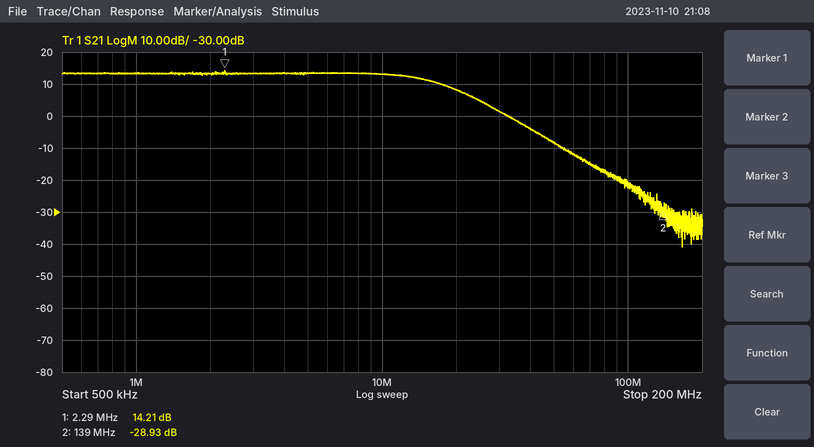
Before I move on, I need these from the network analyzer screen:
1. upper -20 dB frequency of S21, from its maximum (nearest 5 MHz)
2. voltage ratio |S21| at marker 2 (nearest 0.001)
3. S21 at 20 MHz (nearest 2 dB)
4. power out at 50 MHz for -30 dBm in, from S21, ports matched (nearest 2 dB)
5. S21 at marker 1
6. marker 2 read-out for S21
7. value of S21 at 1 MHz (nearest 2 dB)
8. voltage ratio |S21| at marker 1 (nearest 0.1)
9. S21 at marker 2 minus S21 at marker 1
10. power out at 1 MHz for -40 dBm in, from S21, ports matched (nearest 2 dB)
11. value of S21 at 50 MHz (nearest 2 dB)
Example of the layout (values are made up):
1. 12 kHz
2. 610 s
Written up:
1. 45 MHz
2. 0.036
3. 8 dB
4. -38 dBm
5. 14.21 dB
6. -28.93 dB
7. 14 dB
8. 5.1
9. -43.14 dB
10. -26 dBm
11. -8 dB
